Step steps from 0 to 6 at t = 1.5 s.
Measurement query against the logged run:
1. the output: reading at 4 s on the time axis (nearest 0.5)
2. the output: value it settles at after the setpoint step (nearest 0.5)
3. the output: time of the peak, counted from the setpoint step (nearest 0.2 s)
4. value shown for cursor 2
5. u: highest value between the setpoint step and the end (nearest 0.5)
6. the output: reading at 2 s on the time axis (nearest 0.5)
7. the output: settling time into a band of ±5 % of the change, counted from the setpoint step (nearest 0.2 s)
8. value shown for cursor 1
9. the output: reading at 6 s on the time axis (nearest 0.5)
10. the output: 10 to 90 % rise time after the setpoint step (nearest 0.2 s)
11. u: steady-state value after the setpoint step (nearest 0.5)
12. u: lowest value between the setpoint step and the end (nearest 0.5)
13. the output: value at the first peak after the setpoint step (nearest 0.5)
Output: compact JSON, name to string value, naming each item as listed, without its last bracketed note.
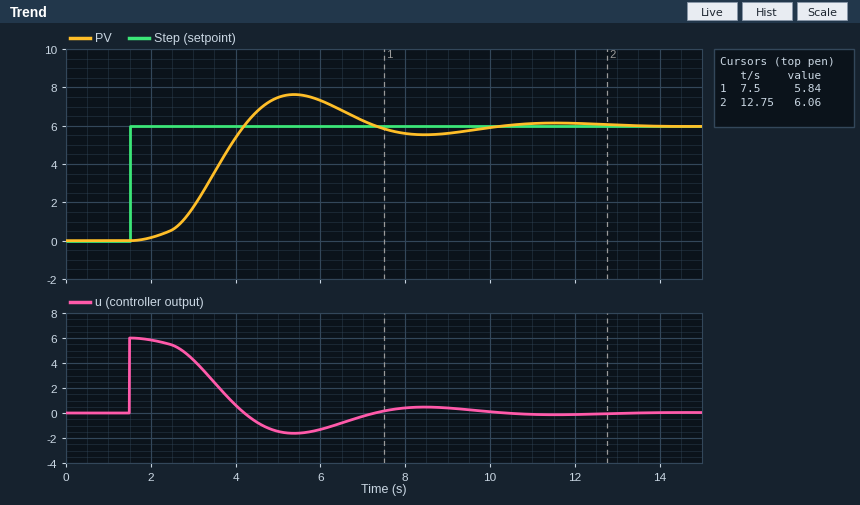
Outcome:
{"the output: reading at 4 s on the time axis": "5.5", "the output: value it settles at after the setpoint step": "6.0", "the output: time of the peak, counted from the setpoint step": "3.8 s", "value shown for cursor 2": "6.06", "u: highest value between the setpoint step and the end": "6.0", "the output: reading at 2 s on the time axis": "0.0", "the output: settling time into a band of ±5 % of the change, counted from the setpoint step": "7.8 s", "value shown for cursor 1": "5.84", "the output: reading at 6 s on the time axis": "7.5", "the output: 10 to 90 % rise time after the setpoint step": "1.4 s", "u: steady-state value after the setpoint step": "0.0", "u: lowest value between the setpoint step and the end": "-1.5", "the output: value at the first peak after the setpoint step": "7.5"}
